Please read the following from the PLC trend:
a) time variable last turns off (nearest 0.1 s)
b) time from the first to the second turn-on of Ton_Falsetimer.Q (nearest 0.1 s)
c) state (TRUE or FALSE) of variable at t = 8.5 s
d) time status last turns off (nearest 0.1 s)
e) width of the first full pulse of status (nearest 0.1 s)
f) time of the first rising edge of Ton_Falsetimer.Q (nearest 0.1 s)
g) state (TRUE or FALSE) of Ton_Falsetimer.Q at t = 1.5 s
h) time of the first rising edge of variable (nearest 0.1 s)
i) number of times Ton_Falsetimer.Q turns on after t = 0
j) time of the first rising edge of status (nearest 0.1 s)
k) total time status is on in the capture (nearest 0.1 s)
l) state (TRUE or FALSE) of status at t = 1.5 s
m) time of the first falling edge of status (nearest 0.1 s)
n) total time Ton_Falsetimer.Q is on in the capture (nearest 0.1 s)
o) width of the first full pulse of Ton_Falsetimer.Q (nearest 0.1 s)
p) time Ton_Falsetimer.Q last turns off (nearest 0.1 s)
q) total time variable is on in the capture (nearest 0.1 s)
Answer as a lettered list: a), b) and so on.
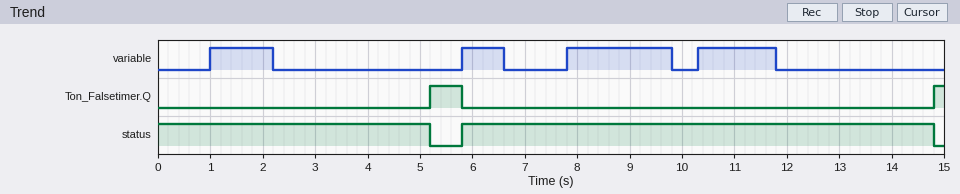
a) 11.8 s
b) 9.6 s
c) TRUE
d) 14.8 s
e) 9.0 s
f) 5.2 s
g) FALSE
h) 1.0 s
i) 2
j) 5.8 s
k) 14.2 s
l) TRUE
m) 5.2 s
n) 0.8 s
o) 0.6 s
p) 5.8 s
q) 5.5 s
